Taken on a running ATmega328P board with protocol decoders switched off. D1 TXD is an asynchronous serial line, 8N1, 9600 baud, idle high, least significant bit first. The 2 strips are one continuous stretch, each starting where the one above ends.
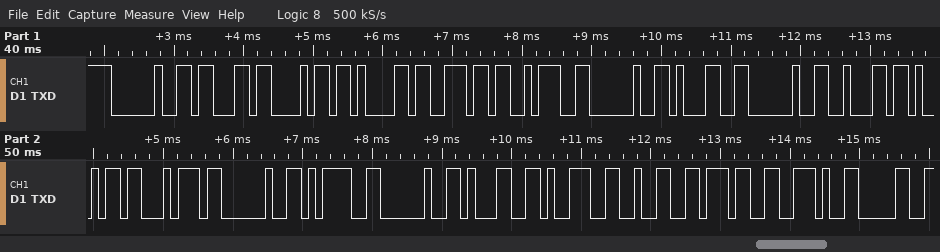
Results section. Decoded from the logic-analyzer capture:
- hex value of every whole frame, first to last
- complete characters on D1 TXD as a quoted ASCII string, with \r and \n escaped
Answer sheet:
20 63 68 61 6E 3A 20 31 20 62 69 74 20 3D 20 31 39 32 37 2E 30
" chan: 1 bit = 1927.0"
